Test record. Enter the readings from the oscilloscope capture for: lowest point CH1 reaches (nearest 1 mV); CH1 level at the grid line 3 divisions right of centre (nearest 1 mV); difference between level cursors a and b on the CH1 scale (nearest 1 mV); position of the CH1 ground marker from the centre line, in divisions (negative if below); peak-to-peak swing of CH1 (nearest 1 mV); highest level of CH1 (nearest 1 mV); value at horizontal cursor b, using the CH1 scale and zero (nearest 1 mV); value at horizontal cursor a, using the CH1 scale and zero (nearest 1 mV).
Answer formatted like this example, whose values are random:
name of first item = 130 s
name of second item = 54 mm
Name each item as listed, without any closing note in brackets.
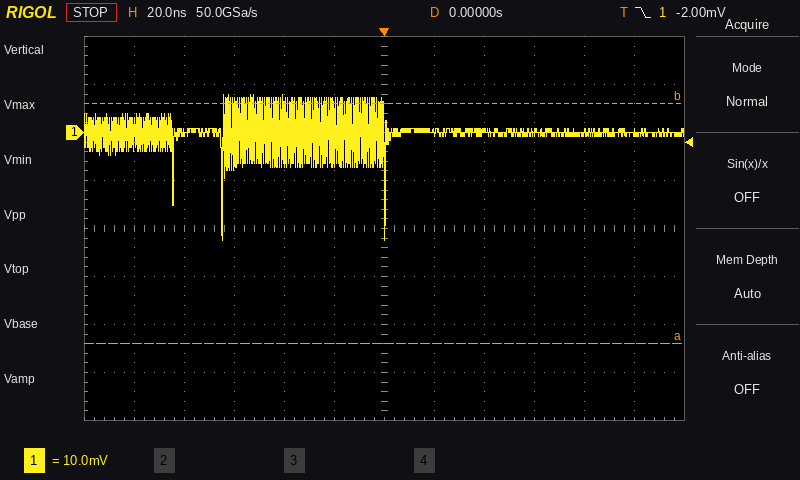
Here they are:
lowest point CH1 reaches = -22 mV
CH1 level at the grid line 3 divisions right of centre = 0 mV
difference between level cursors a and b on the CH1 scale = 50 mV
position of the CH1 ground marker from the centre line, in divisions = +2.0 div
peak-to-peak swing of CH1 = 30 mV
highest level of CH1 = 8 mV
value at horizontal cursor b, using the CH1 scale and zero = 6 mV
value at horizontal cursor a, using the CH1 scale and zero = -44 mV
